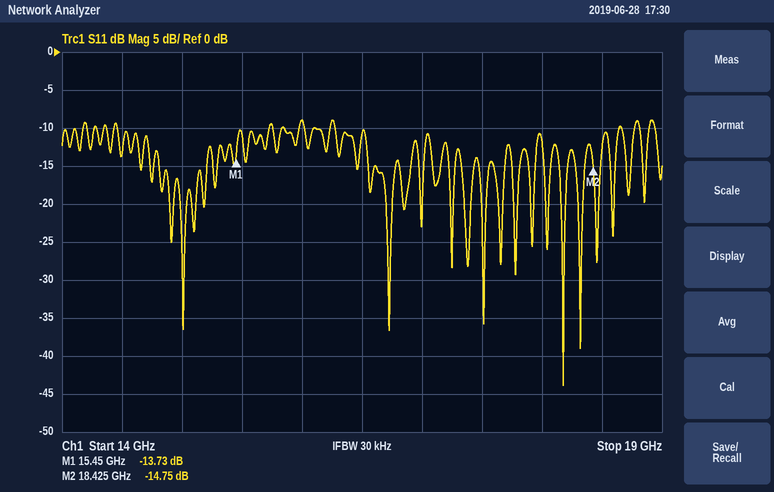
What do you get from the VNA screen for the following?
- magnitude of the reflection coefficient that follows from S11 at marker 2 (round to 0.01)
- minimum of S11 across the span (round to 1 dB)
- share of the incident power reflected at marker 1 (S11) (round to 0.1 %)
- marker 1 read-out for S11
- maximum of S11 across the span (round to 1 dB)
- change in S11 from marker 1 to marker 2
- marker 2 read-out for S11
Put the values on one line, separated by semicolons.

0.18; -44 dB; 4.2 %; -13.73 dB; -9 dB; -1.02 dB; -14.75 dB
